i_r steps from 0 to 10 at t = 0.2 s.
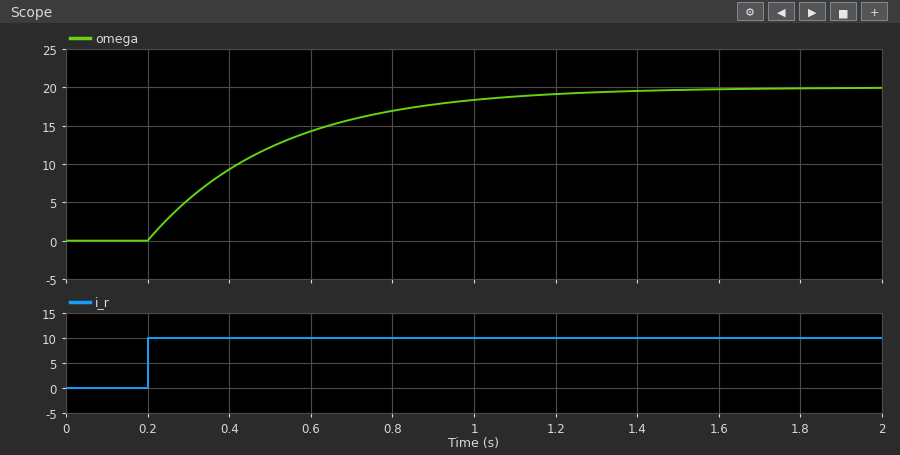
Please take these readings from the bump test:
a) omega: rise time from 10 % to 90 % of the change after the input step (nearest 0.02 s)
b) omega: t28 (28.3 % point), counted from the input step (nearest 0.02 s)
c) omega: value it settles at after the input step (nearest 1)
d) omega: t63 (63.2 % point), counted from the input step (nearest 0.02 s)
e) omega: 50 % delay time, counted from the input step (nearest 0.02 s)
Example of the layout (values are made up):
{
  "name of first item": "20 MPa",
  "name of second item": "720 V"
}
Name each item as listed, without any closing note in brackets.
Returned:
{
  "omega: rise time from 10 % to 90 % of the change after the input step": "0.70 s",
  "omega: t28 (28.3 % point), counted from the input step": "0.10 s",
  "omega: value it settles at after the input step": "20",
  "omega: t63 (63.2 % point), counted from the input step": "0.32 s",
  "omega: 50 % delay time, counted from the input step": "0.22 s"
}
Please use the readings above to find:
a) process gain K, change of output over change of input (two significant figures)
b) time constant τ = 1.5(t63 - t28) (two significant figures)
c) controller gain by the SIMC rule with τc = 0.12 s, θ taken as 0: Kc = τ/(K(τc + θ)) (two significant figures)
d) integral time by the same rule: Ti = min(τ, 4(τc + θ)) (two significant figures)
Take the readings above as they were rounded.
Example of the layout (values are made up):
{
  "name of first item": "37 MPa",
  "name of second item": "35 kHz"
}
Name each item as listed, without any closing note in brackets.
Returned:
{
  "process gain K, change of output over change of input": "2.0",
  "time constant τ = 1.5(t63 - t28)": "0.33 s",
  "controller gain by the SIMC rule with τc = 0.12 s, θ taken as 0: Kc = τ/(K(τc + θ))": "1.4",
  "integral time by the same rule: Ti = min(τ, 4(τc + θ))": "0.33 s"
}
